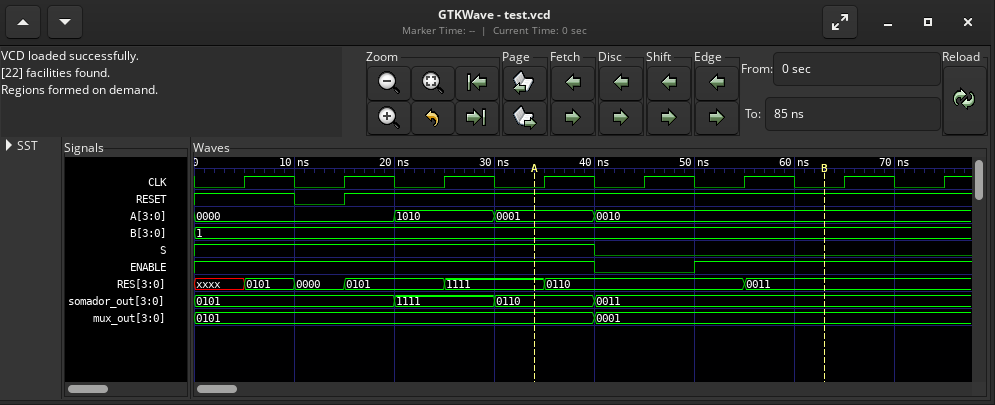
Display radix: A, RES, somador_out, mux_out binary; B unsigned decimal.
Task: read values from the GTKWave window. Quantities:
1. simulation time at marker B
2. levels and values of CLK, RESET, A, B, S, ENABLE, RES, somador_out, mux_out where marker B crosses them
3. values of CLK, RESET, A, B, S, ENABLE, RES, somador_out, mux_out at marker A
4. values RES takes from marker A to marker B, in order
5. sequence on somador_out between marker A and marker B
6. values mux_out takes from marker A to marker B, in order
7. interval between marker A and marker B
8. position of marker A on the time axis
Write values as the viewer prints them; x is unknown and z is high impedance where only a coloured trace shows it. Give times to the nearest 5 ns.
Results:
65 ns
CLK=0, RESET=1, A=0010, B=1, S=0, ENABLE=1, RES=0011, somador_out=0011, mux_out=0001
CLK=0, RESET=1, A=0001, B=1, S=1, ENABLE=1, RES=1111, somador_out=0110, mux_out=0101
1111, 0110, 0011
0110, 0011
0101, 0001
30 ns
35 ns
